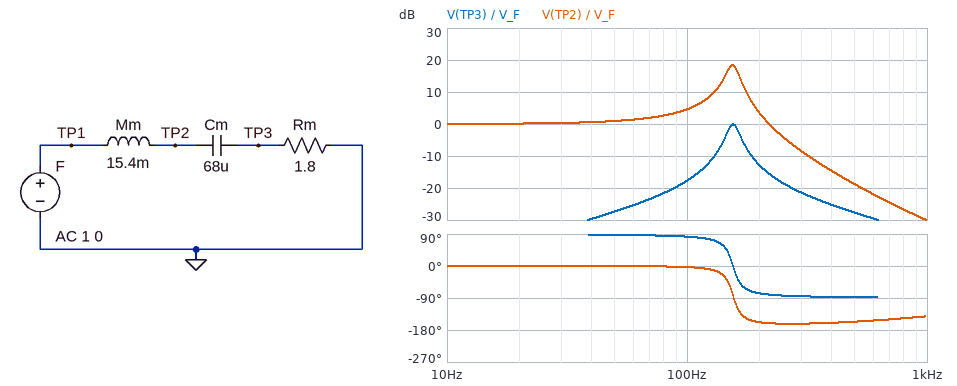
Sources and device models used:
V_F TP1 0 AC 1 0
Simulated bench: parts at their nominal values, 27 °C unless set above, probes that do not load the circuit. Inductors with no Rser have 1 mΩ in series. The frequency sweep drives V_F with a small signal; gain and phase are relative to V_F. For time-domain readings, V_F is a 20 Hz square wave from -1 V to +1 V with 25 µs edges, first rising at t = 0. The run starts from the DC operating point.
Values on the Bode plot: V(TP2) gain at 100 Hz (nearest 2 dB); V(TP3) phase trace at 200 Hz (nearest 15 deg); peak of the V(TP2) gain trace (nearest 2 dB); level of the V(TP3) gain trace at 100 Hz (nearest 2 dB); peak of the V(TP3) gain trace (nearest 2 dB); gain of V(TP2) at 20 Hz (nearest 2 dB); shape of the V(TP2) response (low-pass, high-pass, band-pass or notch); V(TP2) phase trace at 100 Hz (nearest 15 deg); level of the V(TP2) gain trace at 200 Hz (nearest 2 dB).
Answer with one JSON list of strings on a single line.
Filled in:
["4 dB", "-75 deg", "18 dB", "-18 dB", "0 dB", "0 dB", "low-pass", "0 deg", "4 dB"]
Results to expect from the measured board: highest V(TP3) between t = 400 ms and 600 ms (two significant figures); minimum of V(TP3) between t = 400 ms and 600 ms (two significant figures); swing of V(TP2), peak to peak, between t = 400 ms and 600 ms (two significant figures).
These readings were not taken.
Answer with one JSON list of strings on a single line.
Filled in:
["190 mV", "-190 mV", "4.9 V"]
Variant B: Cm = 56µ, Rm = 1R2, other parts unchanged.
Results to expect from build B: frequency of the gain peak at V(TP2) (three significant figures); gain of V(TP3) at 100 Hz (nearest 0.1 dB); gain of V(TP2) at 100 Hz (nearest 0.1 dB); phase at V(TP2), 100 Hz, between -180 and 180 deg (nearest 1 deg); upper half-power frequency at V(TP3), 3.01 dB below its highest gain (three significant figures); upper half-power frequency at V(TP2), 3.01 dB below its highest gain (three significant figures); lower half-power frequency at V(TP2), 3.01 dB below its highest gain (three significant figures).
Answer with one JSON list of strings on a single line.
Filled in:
["171 Hz", "-23.9 dB", "3.6 dB", "-1 deg", "178 Hz", "177 Hz", "165 Hz"]
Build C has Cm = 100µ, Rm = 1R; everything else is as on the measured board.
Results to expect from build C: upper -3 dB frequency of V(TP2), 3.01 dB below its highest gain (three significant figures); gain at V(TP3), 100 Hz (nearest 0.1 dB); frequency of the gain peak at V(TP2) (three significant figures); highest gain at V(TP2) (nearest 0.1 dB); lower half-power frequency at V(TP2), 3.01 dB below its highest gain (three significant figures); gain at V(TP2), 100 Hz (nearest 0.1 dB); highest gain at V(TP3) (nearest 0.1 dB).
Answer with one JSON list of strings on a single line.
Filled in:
["133 Hz", "-16.0 dB", "128 Hz", "21.9 dB", "123 Hz", "8.0 dB", "0 dB"]
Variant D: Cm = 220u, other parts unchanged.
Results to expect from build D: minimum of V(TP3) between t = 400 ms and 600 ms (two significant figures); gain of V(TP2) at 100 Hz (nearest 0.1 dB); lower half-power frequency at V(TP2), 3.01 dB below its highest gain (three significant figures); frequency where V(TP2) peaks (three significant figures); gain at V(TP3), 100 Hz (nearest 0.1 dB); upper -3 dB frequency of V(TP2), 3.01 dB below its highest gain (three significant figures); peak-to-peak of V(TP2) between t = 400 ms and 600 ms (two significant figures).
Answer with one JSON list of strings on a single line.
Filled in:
["-310 mV", "7.8 dB", "75.6 Hz", "85.5 Hz", "-4.5 dB", "94.4 Hz", "4.5 V"]
